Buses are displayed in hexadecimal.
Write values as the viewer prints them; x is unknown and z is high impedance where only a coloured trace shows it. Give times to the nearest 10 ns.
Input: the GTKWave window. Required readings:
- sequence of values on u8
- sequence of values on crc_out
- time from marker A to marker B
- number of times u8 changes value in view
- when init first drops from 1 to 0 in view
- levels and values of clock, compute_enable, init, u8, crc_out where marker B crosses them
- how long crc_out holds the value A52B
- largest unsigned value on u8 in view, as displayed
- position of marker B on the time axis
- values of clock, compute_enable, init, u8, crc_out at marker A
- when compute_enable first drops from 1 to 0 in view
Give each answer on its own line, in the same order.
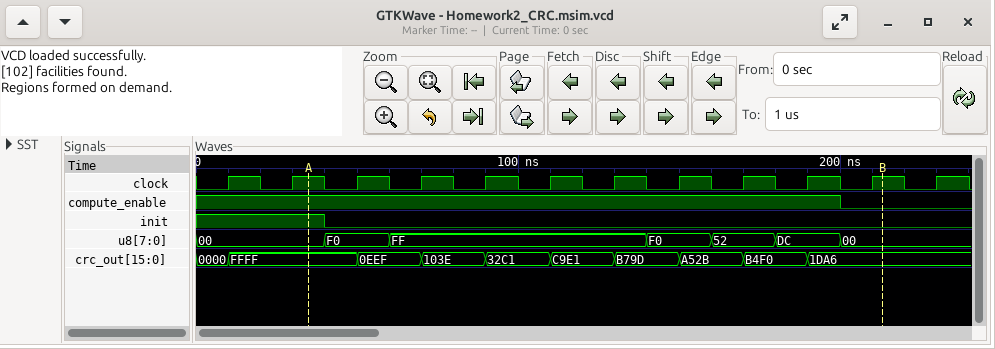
00, F0, FF, F0, 52, DC, 00
0000, FFFF, 0EEF, 103E, 32C1, C9E1, B79D, A52B, B4F0, 1DA6
180 ns
6
40 ns
clock=1, compute_enable=0, init=0, u8=00, crc_out=1DA6
20 ns
FF
210 ns
clock=1, compute_enable=1, init=1, u8=00, crc_out=FFFF
200 ns
